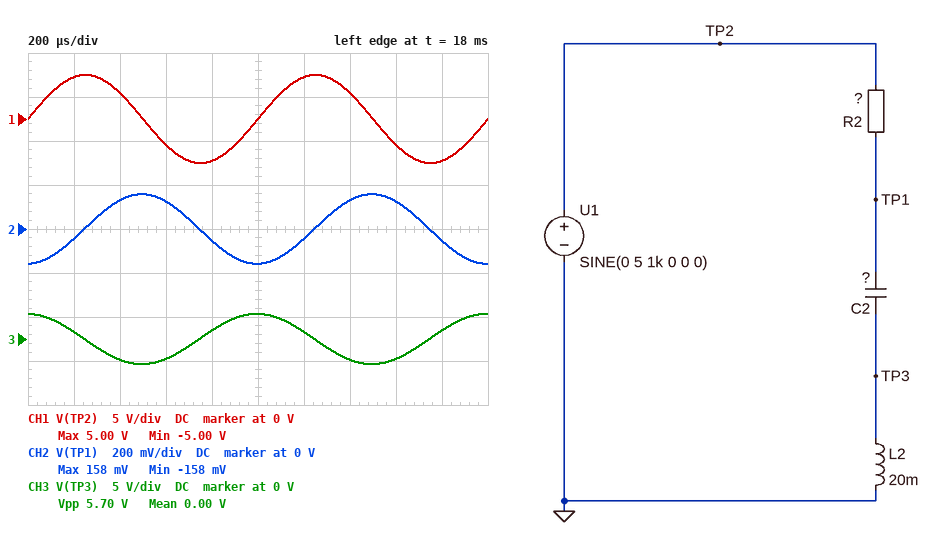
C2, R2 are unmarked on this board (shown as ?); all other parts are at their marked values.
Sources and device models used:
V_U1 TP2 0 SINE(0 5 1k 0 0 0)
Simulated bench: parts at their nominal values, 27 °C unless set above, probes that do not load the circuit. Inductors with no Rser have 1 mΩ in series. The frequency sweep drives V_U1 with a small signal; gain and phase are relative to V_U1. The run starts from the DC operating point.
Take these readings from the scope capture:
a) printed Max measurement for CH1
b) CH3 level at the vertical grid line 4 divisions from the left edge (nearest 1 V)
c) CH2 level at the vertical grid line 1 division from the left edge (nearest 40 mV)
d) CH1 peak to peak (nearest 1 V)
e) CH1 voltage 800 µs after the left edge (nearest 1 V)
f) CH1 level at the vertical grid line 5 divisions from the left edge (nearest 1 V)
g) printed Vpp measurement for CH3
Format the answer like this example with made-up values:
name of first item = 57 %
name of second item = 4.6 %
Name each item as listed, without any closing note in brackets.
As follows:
printed Max measurement for CH1 = 5.00 V
CH3 level at the vertical grid line 4 divisions from the left edge = 1 V
CH2 level at the vertical grid line 1 division from the left edge = -40 mV
CH1 peak to peak = 10 V
CH1 voltage 800 µs after the left edge = -5 V
CH1 level at the vertical grid line 5 divisions from the left edge = 0 V
printed Vpp measurement for CH3 = 5.70 V
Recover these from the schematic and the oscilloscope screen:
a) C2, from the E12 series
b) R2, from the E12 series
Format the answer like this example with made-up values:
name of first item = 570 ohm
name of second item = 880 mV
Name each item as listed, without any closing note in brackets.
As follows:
C2, from the E12 series = 1.2 µF
R2, from the E12 series = 220 Ω
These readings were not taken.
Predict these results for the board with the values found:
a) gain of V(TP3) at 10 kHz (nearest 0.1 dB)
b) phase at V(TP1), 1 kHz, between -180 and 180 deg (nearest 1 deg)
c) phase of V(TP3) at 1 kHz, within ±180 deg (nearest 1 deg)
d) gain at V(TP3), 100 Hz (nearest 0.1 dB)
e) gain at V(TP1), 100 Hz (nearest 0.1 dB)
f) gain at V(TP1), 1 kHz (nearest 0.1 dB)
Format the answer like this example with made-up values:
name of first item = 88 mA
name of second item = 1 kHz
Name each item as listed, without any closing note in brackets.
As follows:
gain of V(TP3) at 10 kHz = 0 dB
phase at V(TP1), 1 kHz, between -180 and 180 deg = -88 deg
phase of V(TP3) at 1 kHz, within ±180 deg = 92 deg
gain at V(TP3), 100 Hz = -40.5 dB
gain at V(TP1), 100 Hz = -0.1 dB
gain at V(TP1), 1 kHz = -30.0 dB
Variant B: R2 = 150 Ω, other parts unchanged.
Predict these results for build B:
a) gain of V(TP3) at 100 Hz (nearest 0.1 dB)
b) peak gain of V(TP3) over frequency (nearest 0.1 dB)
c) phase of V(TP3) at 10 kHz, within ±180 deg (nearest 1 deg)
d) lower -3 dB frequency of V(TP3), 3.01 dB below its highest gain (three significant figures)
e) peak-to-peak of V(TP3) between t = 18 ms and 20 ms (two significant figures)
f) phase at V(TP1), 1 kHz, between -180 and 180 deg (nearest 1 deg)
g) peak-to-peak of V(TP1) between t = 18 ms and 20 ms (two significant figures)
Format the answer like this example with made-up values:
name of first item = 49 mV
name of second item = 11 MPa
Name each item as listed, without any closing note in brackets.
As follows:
gain of V(TP3) at 100 Hz = -40.4 dB
peak gain of V(TP3) over frequency = 0.5 dB
phase of V(TP3) at 10 kHz, within ±180 deg = 7 deg
lower -3 dB frequency of V(TP3), 3.01 dB below its highest gain = 911 Hz
peak-to-peak of V(TP3) between t = 18 ms and 20 ms = 8.4 V
phase at V(TP1), 1 kHz, between -180 and 180 deg = -87 deg
peak-to-peak of V(TP1) between t = 18 ms and 20 ms = 460 mV
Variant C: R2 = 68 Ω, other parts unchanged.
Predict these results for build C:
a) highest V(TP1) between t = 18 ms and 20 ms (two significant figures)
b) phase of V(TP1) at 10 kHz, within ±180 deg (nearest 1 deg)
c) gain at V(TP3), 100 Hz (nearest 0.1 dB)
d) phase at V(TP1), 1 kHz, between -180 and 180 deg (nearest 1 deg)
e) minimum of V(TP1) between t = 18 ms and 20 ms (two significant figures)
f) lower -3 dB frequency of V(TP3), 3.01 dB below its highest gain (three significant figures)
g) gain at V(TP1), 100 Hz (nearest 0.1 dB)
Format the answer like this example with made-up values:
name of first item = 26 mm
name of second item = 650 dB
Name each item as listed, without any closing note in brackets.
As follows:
highest V(TP1) between t = 18 ms and 20 ms = 510 mV
phase of V(TP1) at 10 kHz, within ±180 deg = 3 deg
gain at V(TP3), 100 Hz = -40.4 dB
phase at V(TP1), 1 kHz, between -180 and 180 deg = -84 deg
minimum of V(TP1) between t = 18 ms and 20 ms = -510 mV
lower -3 dB frequency of V(TP3), 3.01 dB below its highest gain = 878 Hz
gain at V(TP1), 100 Hz = 0 dB
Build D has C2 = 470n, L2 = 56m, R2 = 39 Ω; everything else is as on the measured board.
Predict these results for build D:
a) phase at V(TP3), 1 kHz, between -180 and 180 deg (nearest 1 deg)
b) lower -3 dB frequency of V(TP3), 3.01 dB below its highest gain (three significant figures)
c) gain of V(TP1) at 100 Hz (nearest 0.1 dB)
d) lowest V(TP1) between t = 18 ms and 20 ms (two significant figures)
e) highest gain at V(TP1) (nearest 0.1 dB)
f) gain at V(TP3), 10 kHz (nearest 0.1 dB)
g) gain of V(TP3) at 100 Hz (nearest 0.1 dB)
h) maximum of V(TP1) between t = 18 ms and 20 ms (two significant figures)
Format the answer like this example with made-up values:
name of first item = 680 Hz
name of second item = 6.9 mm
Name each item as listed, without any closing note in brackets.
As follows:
phase at V(TP3), 1 kHz, between -180 and 180 deg = 71 deg
lower -3 dB frequency of V(TP3), 3.01 dB below its highest gain = 933 Hz
gain of V(TP1) at 100 Hz = 0 dB
lowest V(TP1) between t = 18 ms and 20 ms = -1.6 V
highest gain at V(TP1) = 0 dB
gain at V(TP3), 10 kHz = 0.1 dB
gain of V(TP3) at 100 Hz = -39.6 dB
maximum of V(TP1) between t = 18 ms and 20 ms = 1.6 V
